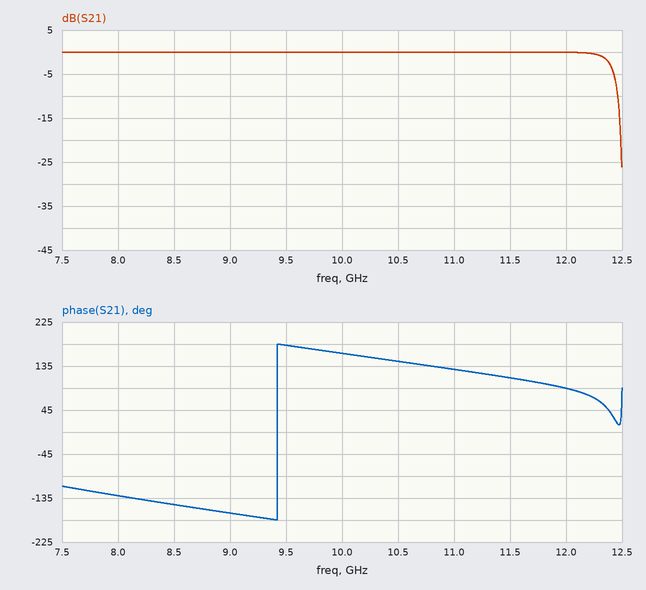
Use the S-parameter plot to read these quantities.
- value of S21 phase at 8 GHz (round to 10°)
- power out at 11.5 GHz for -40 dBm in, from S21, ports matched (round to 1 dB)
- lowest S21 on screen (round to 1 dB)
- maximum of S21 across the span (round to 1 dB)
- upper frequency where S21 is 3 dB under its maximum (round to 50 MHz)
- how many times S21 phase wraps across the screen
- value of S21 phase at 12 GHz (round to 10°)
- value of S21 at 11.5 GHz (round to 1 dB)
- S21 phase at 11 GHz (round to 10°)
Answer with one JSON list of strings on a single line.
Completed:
["-130°", "-40 dBm", "-26 dB", "0 dB", "12.40 GHz", "1", "90°", "0 dB", "130°"]
